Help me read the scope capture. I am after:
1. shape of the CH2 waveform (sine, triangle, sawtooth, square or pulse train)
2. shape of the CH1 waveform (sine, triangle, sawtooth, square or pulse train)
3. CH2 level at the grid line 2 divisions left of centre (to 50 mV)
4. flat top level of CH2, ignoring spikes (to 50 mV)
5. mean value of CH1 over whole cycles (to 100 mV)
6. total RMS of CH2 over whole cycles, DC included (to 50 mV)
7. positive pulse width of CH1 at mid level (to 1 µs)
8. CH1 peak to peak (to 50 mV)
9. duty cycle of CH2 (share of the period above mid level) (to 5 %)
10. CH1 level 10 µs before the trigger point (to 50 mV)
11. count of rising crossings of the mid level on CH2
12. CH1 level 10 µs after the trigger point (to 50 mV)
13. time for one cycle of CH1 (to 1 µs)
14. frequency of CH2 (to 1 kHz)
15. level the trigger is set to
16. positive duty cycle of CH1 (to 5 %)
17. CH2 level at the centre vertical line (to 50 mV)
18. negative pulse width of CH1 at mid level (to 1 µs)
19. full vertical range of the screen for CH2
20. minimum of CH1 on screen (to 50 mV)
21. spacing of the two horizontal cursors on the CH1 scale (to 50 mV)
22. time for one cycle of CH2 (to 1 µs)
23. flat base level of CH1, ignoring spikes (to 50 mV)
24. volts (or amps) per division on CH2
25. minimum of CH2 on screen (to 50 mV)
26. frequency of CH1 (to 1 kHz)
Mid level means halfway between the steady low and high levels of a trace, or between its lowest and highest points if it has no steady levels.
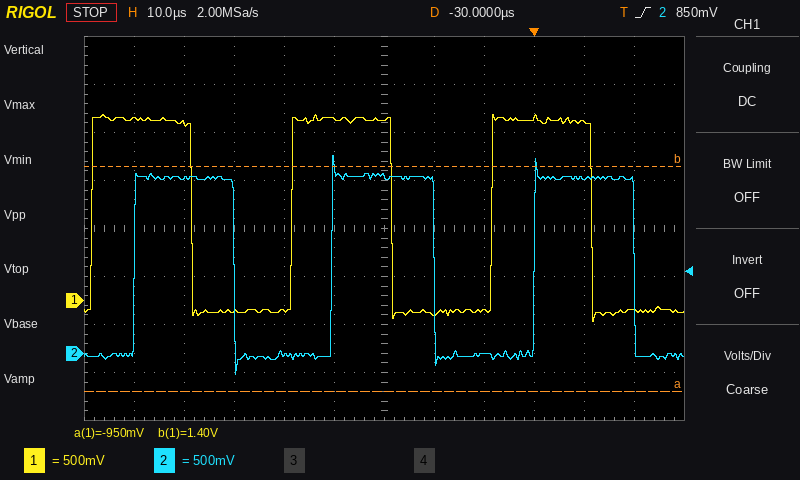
square
square
0 mV
1.85 V
900 mV
1.30 V
20 µs
2.15 V
50 %
-100 mV
3
1.85 V
40 µs
25 kHz
850 mV
50 %
1.85 V
20 µs
4 V
-200 mV
2.35 V
40 µs
-100 mV
500 mV
-200 mV
25 kHz
